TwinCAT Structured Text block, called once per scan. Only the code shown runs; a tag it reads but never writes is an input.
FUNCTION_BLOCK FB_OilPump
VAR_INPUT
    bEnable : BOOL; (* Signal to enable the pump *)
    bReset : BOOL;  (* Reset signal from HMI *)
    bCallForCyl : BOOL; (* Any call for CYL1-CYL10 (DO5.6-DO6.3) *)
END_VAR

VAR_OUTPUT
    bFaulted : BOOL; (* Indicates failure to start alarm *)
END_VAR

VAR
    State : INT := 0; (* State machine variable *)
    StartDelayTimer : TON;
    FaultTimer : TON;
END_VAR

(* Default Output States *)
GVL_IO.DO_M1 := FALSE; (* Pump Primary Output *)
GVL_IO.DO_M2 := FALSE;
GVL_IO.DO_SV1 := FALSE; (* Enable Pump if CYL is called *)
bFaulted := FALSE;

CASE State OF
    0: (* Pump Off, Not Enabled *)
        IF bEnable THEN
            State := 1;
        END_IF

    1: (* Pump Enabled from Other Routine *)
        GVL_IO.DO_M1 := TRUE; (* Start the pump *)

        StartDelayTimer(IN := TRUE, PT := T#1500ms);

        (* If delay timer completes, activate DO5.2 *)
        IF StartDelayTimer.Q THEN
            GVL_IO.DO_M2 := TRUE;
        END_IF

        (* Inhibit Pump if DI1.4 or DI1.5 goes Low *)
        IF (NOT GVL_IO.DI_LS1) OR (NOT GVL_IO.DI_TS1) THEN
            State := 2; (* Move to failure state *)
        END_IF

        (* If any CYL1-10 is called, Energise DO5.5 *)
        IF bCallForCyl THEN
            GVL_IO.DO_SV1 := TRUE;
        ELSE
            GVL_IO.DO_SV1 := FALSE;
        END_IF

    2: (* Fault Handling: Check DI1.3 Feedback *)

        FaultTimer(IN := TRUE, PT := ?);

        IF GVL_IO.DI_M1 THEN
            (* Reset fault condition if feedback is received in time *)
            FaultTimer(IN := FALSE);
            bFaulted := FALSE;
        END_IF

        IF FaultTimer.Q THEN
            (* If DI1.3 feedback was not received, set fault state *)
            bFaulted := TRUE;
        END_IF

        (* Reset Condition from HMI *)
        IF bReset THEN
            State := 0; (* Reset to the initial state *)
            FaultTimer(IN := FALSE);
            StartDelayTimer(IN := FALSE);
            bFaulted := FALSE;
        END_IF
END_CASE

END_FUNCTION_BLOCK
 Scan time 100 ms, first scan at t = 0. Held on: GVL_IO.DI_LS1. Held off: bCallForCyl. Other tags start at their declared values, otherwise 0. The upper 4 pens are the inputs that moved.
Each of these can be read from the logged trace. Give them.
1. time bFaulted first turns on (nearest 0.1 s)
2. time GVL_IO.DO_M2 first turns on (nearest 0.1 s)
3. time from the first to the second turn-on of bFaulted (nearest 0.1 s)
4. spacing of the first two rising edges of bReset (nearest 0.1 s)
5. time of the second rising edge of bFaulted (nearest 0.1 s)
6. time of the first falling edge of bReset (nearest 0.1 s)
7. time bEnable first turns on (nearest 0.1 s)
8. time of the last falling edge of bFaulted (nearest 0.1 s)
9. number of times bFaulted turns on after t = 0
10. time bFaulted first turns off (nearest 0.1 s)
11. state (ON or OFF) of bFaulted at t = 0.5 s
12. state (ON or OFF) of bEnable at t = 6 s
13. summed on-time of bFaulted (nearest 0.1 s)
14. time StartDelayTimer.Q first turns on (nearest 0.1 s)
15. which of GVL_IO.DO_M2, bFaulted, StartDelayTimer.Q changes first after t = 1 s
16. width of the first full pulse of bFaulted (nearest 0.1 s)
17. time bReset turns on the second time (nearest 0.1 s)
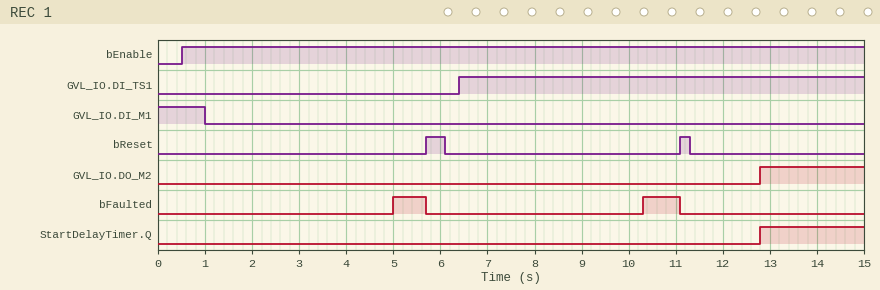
5.0 s
12.8 s
5.3 s
5.4 s
10.3 s
6.1 s
0.5 s
11.1 s
2
5.7 s
OFF
ON
1.5 s
12.8 s
bFaulted
0.7 s
11.1 s
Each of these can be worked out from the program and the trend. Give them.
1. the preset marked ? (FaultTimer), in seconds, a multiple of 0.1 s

4.0 s
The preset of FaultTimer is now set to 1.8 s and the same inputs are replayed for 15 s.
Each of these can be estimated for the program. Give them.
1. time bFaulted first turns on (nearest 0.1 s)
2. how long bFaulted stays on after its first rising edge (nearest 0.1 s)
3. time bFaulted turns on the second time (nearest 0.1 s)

2.8 s
2.9 s
8.1 s
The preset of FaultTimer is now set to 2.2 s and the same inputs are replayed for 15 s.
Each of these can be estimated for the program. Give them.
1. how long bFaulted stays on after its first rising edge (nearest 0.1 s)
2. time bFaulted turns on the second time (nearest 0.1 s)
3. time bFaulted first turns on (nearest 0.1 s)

2.5 s
8.5 s
3.2 s
